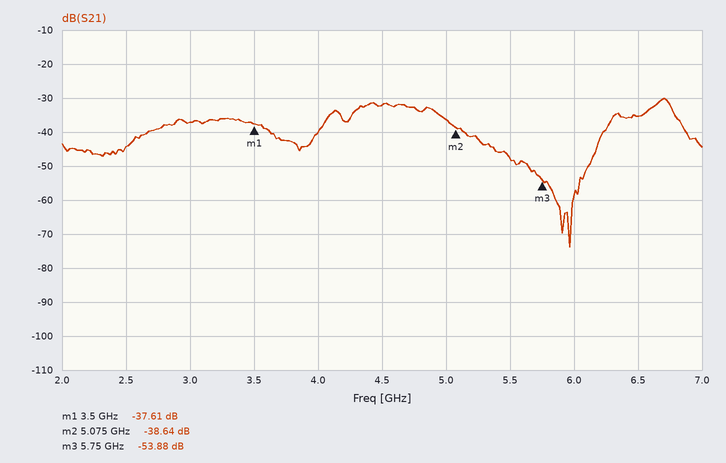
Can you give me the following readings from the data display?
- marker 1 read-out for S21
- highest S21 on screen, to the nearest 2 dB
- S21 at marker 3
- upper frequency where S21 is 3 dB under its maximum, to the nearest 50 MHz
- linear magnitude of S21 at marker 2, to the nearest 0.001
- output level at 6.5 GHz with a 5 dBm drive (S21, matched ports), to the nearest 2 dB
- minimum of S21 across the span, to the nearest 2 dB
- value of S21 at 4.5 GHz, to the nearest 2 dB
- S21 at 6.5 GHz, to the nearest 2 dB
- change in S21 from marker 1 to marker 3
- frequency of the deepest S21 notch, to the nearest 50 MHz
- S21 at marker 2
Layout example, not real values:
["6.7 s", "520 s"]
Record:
["-37.61 dB", "-30 dB", "-53.88 dB", "6.75 GHz", "0.012", "-30 dBm", "-74 dB", "-32 dB", "-36 dB", "-16.27 dB", "5.95 GHz", "-38.64 dB"]
